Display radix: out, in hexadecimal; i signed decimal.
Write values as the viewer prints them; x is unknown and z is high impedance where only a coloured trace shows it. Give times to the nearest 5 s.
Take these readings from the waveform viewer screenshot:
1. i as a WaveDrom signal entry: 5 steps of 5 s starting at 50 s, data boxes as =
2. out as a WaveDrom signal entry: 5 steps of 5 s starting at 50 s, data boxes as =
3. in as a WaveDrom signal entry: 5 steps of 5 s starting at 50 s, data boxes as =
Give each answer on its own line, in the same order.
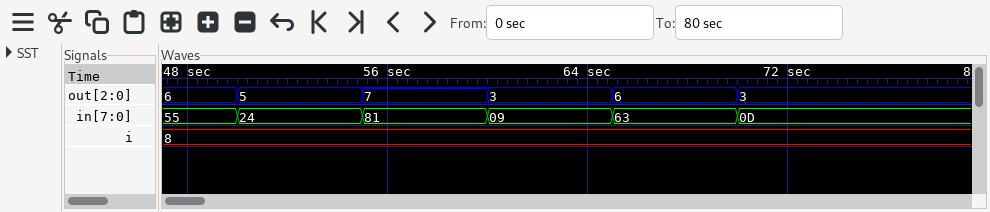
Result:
{name: 'i', wave: '=....', data: '8'}
{name: 'out', wave: '=====', data: '5 7 3 6 3'}
{name: 'in', wave: '=====', data: '24 81 09 63 0D'}
